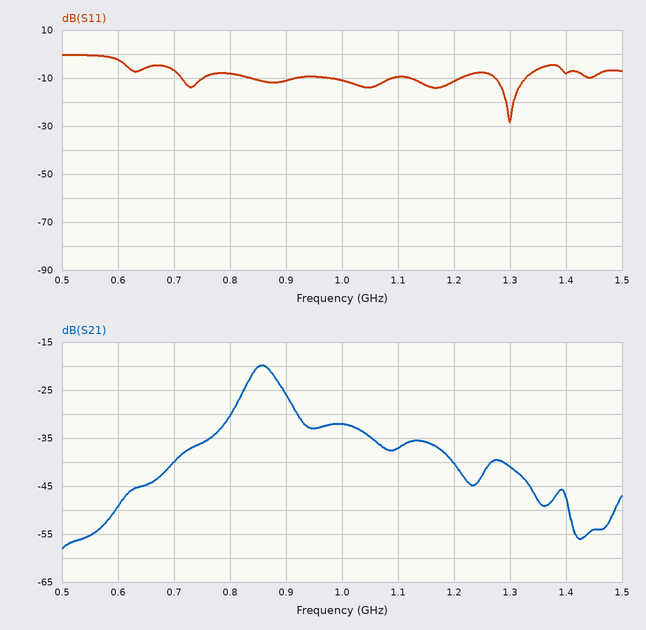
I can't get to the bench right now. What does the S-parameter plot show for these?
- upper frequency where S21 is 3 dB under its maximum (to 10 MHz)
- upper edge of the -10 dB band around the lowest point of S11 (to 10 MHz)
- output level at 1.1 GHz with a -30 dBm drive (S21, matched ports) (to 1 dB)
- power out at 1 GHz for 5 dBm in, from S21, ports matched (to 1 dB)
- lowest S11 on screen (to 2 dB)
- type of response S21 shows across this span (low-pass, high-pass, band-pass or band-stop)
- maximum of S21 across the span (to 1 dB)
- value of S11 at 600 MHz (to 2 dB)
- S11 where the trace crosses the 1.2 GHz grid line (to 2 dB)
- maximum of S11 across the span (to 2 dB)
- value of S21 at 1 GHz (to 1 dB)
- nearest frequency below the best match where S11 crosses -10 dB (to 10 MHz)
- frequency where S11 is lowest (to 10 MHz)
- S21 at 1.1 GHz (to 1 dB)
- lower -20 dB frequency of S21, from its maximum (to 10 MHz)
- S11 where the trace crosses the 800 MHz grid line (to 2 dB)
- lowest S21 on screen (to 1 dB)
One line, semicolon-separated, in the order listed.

880 MHz; 1.33 GHz; -67 dBm; -27 dBm; -28 dB; band-pass; -20 dB; -2 dB; -12 dB; 0 dB; -32 dB; 1.27 GHz; 1.30 GHz; -37 dB; 700 MHz; -8 dB; -58 dB
